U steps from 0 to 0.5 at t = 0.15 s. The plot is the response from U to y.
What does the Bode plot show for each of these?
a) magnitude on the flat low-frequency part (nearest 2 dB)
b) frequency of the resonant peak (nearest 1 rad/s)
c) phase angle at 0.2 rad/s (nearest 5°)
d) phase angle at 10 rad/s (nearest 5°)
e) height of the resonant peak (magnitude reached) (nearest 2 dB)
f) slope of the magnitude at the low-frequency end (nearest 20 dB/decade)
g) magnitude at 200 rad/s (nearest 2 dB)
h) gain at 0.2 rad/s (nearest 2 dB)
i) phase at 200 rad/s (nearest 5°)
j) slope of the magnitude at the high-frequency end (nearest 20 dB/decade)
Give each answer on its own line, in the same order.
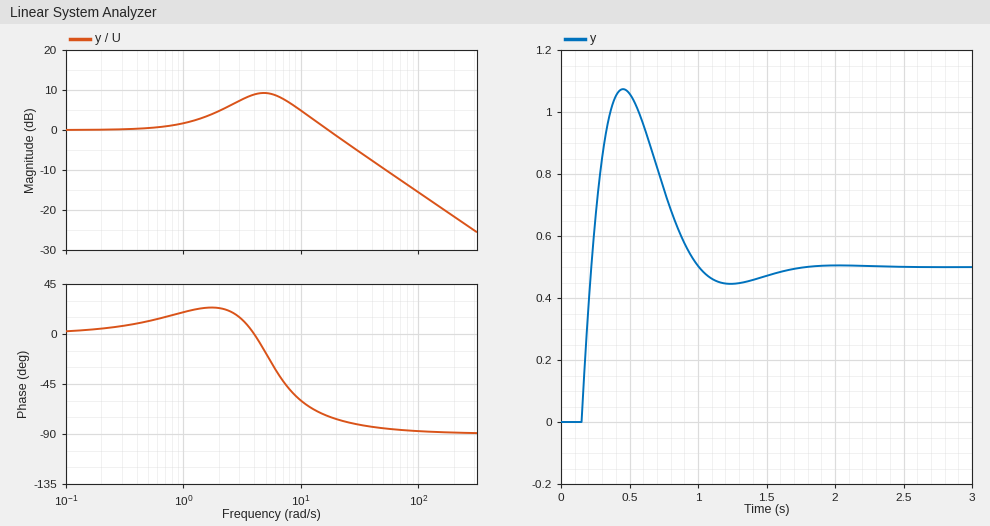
0 dB
5 rad/s
5°
-60°
10 dB
0 dB/decade
-22 dB
0 dB
-90°
-20 dB/decade
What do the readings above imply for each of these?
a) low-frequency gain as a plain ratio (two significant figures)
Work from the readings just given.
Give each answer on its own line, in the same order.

1.0
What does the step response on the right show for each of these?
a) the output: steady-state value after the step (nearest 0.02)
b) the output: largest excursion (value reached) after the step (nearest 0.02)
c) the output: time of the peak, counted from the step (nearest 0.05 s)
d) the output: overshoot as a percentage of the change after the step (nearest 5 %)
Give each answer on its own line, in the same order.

0.50
1.08
0.30 s
115 %
